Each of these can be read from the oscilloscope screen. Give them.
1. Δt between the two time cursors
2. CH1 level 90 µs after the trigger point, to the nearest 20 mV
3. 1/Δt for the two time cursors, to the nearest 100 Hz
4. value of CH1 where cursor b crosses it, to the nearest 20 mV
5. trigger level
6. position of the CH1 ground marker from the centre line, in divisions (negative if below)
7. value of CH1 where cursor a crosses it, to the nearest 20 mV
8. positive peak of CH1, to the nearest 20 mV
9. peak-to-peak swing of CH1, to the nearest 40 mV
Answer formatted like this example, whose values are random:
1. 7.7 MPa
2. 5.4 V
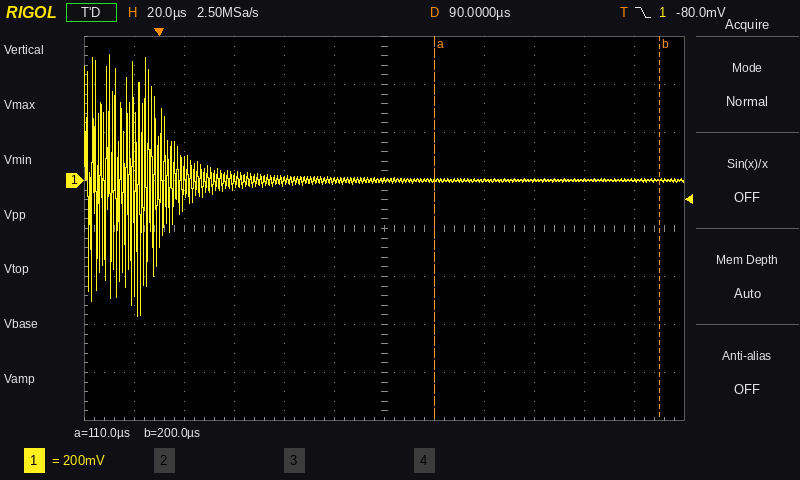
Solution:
1. 90 µs
2. 0 mV
3. 11.1 kHz
4. 0 mV
5. -80.0 mV
6. +1.0 div
7. 0 mV
8. 520 mV
9. 1.08 V
